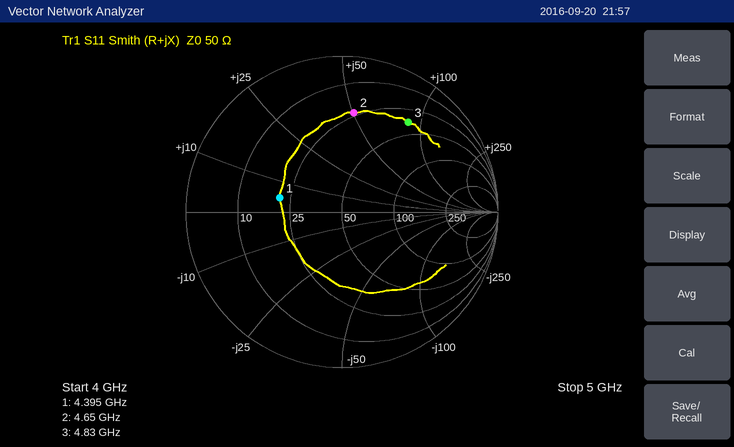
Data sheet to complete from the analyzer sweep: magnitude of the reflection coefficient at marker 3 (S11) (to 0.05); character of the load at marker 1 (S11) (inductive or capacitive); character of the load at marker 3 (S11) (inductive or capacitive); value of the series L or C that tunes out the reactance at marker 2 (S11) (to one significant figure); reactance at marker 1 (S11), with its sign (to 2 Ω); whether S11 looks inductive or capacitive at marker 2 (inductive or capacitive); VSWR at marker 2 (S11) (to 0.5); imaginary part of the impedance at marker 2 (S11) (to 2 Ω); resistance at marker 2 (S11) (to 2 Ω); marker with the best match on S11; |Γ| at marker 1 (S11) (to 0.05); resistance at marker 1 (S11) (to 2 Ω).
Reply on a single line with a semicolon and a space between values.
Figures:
0.70; inductive; inductive; 700 fF; +4 Ω; inductive; 4.5; +50 Ω; 24 Ω; marker 1; 0.40; 22 Ω
